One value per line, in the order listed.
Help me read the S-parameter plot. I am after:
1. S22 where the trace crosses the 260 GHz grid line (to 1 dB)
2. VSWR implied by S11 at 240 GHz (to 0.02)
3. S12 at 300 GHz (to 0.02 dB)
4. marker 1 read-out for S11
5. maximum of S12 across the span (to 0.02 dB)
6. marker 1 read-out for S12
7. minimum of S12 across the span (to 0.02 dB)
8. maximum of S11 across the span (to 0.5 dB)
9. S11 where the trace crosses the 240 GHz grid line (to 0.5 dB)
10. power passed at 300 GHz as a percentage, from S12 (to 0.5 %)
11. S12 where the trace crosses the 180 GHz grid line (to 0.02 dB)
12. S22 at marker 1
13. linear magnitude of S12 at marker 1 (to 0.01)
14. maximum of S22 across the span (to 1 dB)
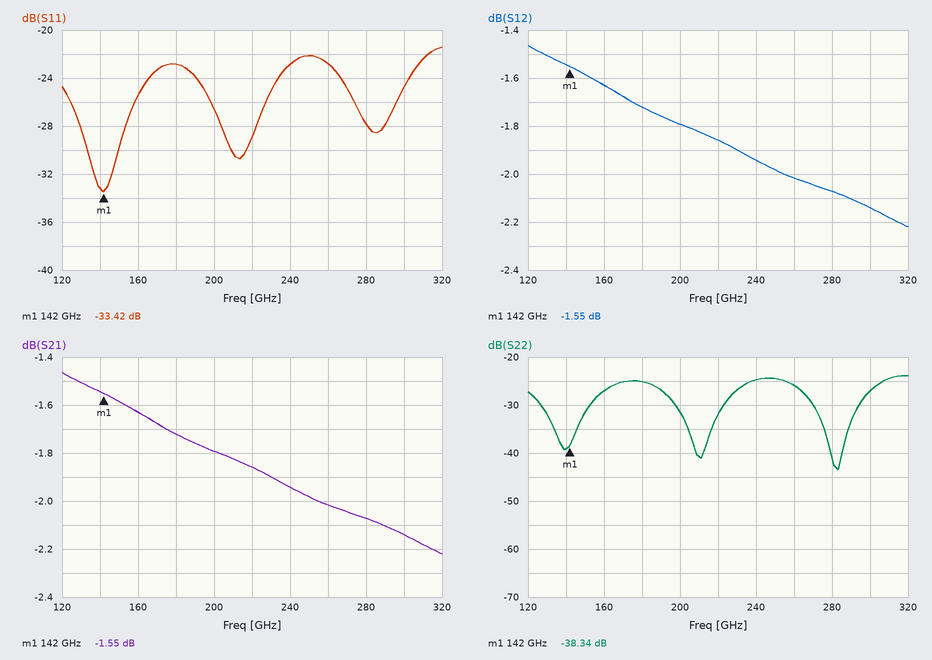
-26 dB
1.16
-2.14 dB
-33.42 dB
-1.46 dB
-1.55 dB
-2.22 dB
-21.5 dB
-23.0 dB
61.0 %
-1.72 dB
-38.34 dB
0.84
-24 dB
